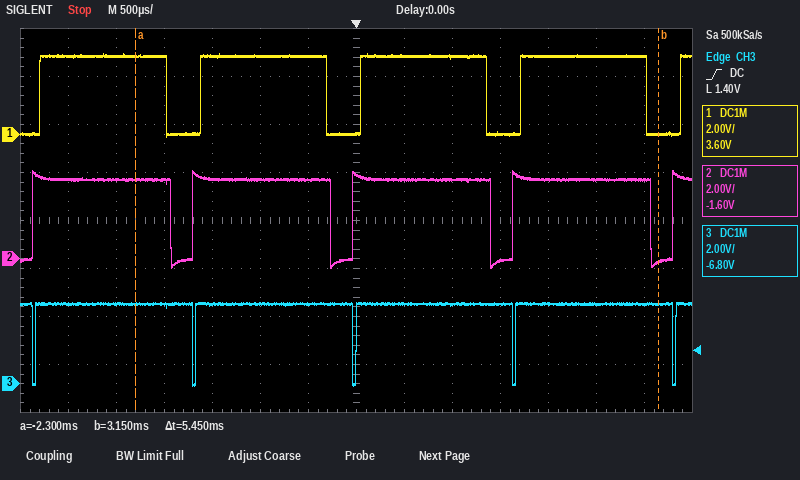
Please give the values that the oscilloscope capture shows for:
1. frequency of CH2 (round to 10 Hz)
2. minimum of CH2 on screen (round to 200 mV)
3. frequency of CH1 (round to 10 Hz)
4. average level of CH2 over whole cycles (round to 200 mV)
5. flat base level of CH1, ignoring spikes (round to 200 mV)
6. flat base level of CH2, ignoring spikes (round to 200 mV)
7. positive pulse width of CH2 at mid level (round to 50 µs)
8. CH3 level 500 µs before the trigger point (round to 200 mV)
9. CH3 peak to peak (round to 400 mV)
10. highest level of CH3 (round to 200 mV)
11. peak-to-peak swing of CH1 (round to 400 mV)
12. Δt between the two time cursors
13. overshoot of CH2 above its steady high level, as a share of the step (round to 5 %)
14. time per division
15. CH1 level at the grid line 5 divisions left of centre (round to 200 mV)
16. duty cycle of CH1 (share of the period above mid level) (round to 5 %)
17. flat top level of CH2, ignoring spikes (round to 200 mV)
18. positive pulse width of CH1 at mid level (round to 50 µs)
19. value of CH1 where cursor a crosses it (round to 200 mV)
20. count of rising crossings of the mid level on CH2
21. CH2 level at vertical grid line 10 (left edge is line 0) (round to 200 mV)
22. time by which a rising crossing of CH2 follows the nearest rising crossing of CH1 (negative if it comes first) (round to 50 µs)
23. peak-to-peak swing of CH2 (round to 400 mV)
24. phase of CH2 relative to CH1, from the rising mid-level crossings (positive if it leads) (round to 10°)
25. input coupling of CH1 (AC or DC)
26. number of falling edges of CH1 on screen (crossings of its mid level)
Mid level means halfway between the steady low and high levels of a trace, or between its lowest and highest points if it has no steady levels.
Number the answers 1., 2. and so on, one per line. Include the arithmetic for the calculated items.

1. 1 / 1.66 ms ≈ 602 Hz, so 600 Hz to the nearest 10 Hz
2. -400 mV
3. 600 Hz
4. 0.0 V + 0.85 × (3.4 V − (0.0 V)) ≈ 2.89 V, so 2.8 V to the nearest 200 mV
5. 0.0 V
6. 0.0 V
7. 1.45 ms
8. 3.4 V
9. 3.6 V
10. 3.4 V
11. 3.6 V
12. 5.45 ms
13. 10 %
14. 500 µs
15. 3.2 V
16. 80 %
17. 3.4 V
18. 1.30 ms
19. 3.2 V
20. 5
21. 0.0 V
22. -100 µs
23. 4.0 V
24. −360° × (-100 µs) / 1.66 ms ≈ +21.7°, so +20° to the nearest 10°
25. DC
26. 4
